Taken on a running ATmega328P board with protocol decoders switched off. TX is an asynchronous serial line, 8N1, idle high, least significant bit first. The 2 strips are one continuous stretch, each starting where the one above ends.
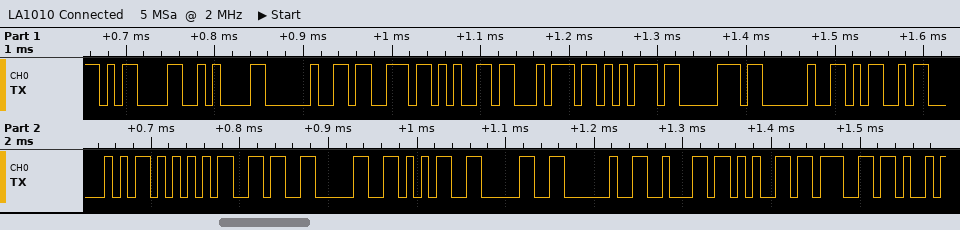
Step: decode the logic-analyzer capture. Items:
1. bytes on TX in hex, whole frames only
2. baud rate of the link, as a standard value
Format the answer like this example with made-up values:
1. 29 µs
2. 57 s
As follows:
1. 0D 0A 20 73 65 74 75 70 20 4D 50 55 36 30 35 30 20 62 65 67
2. 115200 baud
